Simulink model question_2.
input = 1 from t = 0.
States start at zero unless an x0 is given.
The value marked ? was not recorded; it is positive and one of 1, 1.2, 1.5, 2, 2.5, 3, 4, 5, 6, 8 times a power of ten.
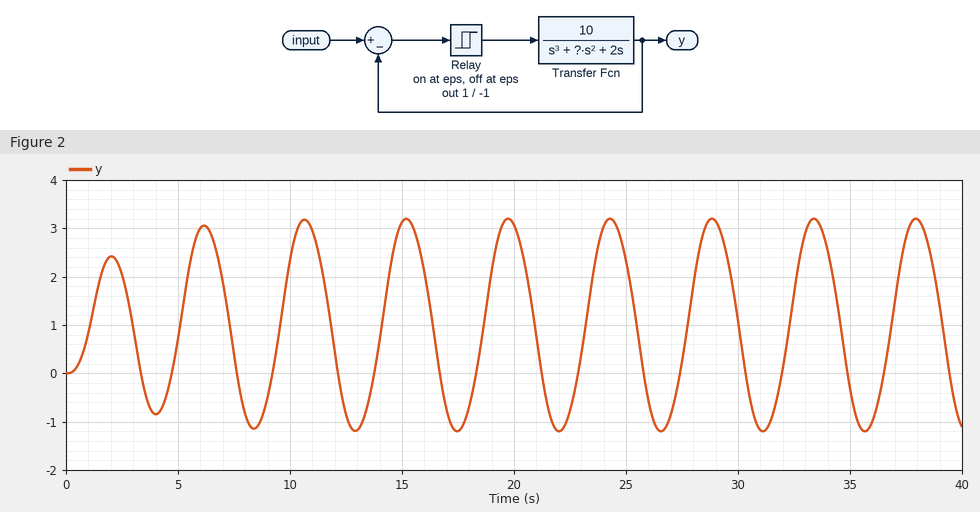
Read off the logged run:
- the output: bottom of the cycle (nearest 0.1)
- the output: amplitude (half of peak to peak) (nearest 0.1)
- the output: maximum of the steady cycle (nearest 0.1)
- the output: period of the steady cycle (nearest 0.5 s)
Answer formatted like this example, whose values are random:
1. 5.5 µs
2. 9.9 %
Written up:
1. -1.2
2. 2.2
3. 3.2
4. 4.5 s
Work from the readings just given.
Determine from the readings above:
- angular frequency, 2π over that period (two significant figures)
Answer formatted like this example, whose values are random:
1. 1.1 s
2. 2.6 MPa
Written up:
1. 1.4 rad/s
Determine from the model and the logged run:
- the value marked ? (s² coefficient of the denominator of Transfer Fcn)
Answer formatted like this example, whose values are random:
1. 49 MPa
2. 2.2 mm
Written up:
1. 3
